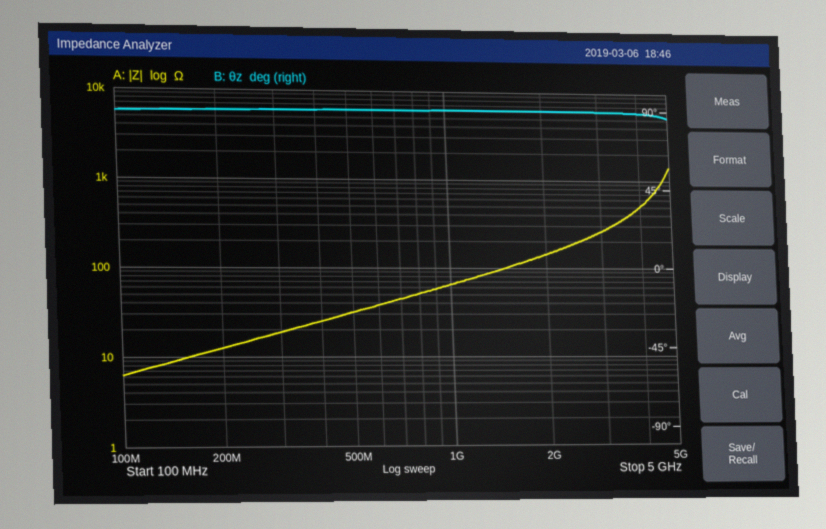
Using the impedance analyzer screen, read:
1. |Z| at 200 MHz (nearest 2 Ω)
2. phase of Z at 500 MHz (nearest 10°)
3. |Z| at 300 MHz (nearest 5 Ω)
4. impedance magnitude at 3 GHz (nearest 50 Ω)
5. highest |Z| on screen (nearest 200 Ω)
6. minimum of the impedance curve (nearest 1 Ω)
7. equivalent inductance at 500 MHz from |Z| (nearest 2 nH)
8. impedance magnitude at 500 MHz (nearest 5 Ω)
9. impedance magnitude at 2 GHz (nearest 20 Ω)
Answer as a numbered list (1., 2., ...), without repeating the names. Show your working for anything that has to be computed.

1. 12 Ω
2. 90°
3. 20 Ω
4. 250 Ω
5. 1.4 kΩ
6. 6 Ω
7. L = 30 Ω/(2π × 500 MHz) ≈ 10 nH
8. 30 Ω
9. 140 Ω
